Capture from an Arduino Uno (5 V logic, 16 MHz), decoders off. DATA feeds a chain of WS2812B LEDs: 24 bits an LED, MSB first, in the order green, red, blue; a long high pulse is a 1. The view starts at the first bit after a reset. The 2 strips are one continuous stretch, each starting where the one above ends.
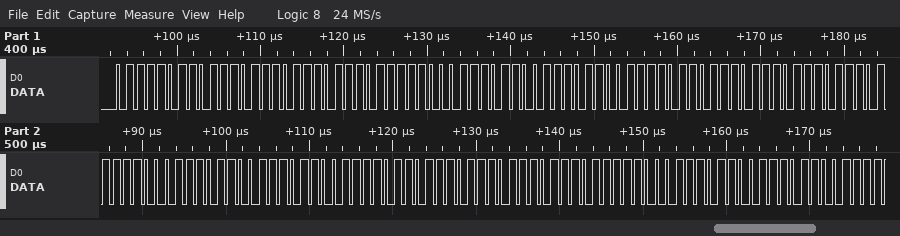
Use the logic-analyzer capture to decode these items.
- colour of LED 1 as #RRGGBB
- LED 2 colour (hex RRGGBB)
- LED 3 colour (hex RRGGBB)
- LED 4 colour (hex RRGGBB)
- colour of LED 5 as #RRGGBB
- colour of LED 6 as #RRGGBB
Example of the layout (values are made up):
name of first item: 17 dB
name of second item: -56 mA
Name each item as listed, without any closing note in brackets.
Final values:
colour of LED 1 as #RRGGBB: #777B77
LED 2 colour: #767C76
LED 3 colour: #777B77
LED 4 colour: #767C76
colour of LED 5 as #RRGGBB: #777B77
colour of LED 6 as #RRGGBB: #767C76
